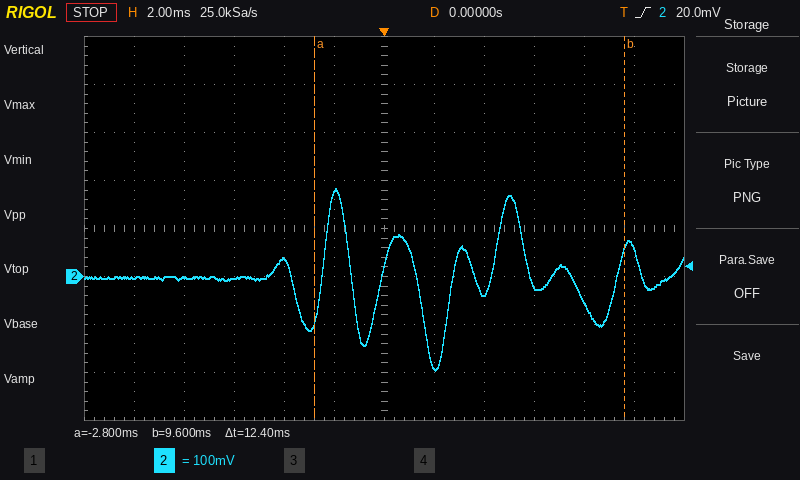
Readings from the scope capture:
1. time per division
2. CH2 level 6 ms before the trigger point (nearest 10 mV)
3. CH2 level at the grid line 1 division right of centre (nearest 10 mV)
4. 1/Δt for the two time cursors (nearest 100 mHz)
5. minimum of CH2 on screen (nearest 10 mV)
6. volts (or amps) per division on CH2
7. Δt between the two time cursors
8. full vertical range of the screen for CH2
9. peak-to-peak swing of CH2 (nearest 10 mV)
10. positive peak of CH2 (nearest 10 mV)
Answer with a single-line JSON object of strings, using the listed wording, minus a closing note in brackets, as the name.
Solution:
{"time per division": "2 ms", "CH2 level 6 ms before the trigger point": "0 mV", "CH2 level at the grid line 1 division right of centre": "-190 mV", "1/Δt for the two time cursors": "80.6 Hz", "minimum of CH2 on screen": "-200 mV", "volts (or amps) per division on CH2": "100 mV", "Δt between the two time cursors": "12.4 ms", "full vertical range of the screen for CH2": "800 mV", "peak-to-peak swing of CH2": "380 mV", "positive peak of CH2": "180 mV"}
